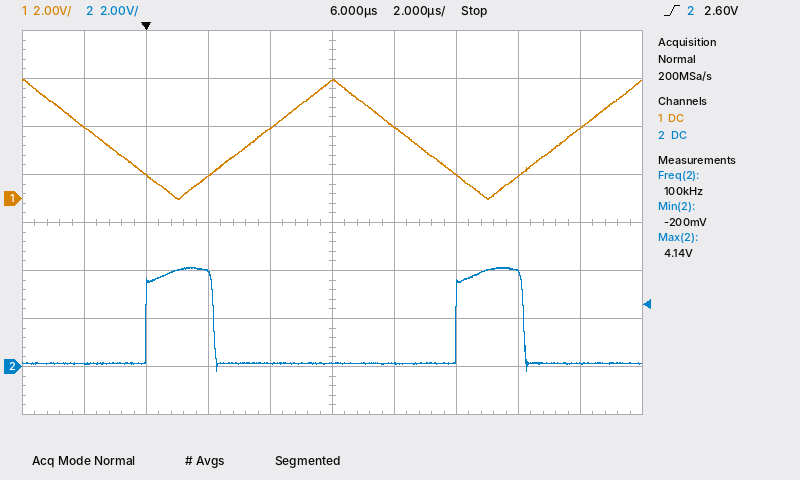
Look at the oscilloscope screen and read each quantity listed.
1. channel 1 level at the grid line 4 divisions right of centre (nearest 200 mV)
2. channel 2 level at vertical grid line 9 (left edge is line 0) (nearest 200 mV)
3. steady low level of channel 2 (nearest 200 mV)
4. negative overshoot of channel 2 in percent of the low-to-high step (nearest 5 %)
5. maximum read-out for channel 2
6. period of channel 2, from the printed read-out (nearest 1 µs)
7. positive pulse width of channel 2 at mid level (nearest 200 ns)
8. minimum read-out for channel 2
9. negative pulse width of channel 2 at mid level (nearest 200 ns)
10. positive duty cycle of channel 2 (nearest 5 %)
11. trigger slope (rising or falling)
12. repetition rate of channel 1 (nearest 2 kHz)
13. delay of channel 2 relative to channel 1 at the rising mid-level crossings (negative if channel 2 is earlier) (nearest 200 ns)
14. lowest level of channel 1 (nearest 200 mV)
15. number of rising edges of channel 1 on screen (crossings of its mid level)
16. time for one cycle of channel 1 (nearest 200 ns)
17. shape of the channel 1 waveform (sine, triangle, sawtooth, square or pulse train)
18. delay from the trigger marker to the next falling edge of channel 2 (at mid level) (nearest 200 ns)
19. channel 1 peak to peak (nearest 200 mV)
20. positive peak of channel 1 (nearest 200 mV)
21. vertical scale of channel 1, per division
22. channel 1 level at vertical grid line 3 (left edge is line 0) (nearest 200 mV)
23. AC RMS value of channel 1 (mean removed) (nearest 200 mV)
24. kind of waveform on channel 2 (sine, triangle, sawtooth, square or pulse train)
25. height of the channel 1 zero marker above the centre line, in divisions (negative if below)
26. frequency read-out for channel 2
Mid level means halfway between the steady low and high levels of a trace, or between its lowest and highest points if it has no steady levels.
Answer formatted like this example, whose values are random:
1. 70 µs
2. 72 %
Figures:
1. 3.0 V
2. 200 mV
3. 200 mV
4. 10 %
5. 4.14 V
6. 10 µs
7. 2.2 µs
8. -200 mV
9. 7.8 µs
10. 20 %
11. rising
12. 100 kHz
13. -3.6 µs
14. 0.0 V
15. 2
16. 10.0 µs
17. triangle
18. 2.2 µs
19. 5.0 V
20. 5.0 V
21. 2 V
22. 1.0 V
23. 1.4 V
24. pulse train
25. +0.5 div
26. 100 kHz
